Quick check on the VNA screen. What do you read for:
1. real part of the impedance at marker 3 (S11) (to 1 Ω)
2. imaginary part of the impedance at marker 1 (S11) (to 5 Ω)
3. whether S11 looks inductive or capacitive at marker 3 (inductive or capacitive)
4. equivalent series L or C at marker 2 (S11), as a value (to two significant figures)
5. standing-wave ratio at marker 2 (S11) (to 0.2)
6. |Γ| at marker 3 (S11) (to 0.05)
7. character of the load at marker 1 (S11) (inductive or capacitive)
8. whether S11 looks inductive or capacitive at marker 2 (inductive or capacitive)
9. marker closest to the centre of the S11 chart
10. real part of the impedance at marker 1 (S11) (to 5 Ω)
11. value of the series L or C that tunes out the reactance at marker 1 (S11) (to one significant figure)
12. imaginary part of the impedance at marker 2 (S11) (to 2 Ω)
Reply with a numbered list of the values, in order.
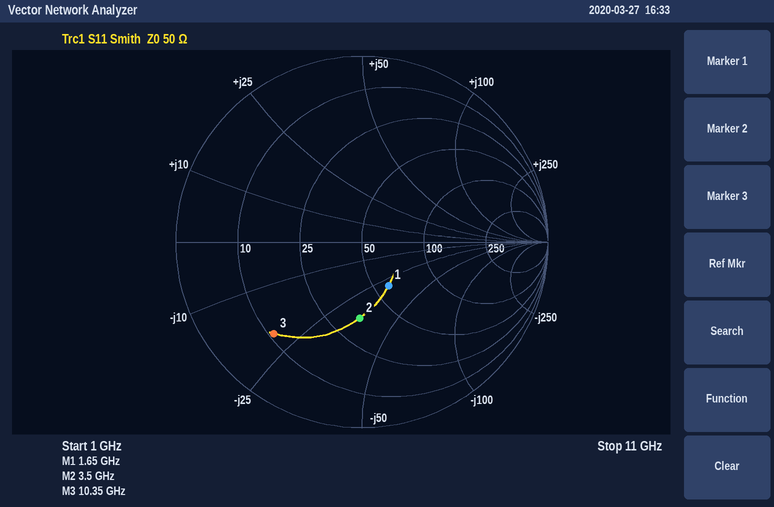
1. 11 Ω
2. -30 Ω
3. capacitive
4. 1.3 pF
5. 2.4
6. 0.70
7. capacitive
8. capacitive
9. marker 1
10. 60 Ω
11. 3 nH
12. -34 Ω
